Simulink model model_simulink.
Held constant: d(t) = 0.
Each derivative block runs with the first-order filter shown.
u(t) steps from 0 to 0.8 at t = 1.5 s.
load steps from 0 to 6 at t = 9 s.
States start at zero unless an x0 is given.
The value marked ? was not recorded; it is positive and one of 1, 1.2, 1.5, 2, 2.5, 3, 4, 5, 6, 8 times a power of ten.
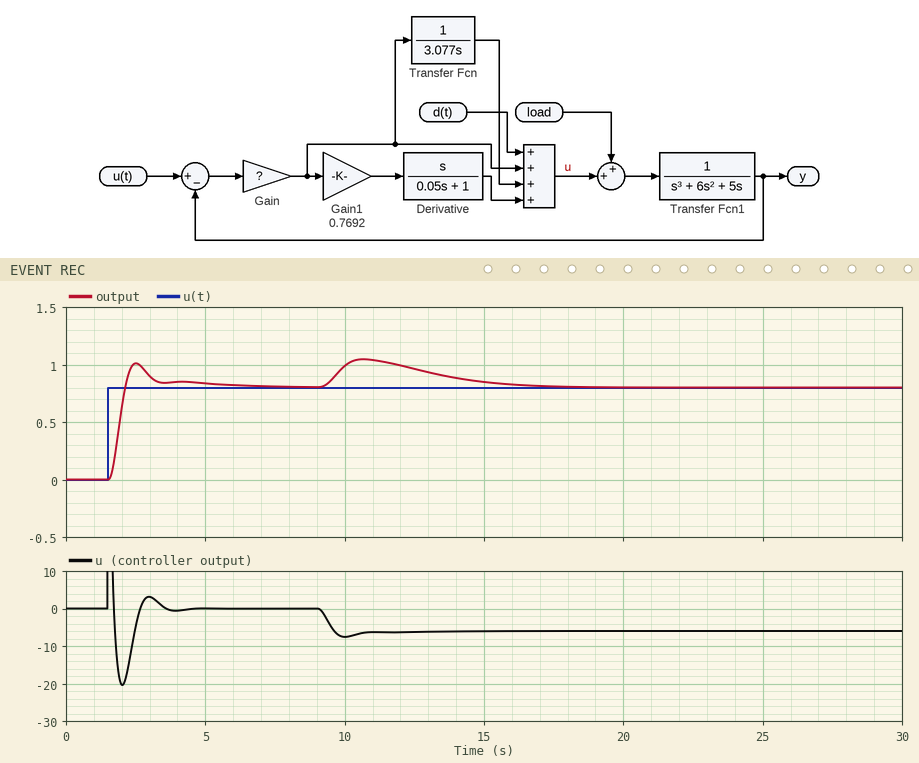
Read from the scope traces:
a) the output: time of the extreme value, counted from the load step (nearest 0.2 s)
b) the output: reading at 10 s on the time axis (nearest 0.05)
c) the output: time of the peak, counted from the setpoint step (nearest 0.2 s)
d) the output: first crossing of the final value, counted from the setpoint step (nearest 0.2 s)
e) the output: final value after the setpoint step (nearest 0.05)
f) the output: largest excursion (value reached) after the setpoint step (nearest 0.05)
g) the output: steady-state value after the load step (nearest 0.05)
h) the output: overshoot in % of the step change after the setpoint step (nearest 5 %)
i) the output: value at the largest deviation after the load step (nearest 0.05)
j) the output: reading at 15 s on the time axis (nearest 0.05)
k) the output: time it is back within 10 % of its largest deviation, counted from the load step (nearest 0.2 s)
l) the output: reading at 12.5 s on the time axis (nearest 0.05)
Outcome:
1.6 s
1.00
1.0 s
0.6 s
0.80
1.00
0.80
25 %
1.05
0.85
7.2 s
0.95
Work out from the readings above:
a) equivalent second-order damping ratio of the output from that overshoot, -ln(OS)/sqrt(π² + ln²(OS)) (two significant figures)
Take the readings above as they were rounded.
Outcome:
0.40
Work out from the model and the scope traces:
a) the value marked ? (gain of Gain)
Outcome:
20
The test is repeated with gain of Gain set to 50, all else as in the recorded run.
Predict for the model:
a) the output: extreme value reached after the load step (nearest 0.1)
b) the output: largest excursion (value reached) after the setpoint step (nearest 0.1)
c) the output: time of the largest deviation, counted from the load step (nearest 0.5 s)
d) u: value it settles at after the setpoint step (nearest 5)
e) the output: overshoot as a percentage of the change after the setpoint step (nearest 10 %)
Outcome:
0.9
1.2
2.0 s
0
50 %
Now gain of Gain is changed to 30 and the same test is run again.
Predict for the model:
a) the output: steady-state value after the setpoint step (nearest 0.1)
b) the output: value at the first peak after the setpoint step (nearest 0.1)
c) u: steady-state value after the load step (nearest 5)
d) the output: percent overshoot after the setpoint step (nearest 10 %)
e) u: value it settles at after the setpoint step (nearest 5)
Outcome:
0.8
1.1
-5
40 %
0
